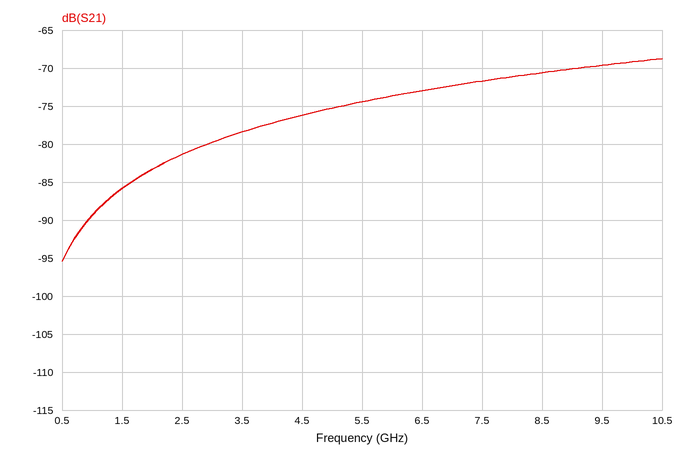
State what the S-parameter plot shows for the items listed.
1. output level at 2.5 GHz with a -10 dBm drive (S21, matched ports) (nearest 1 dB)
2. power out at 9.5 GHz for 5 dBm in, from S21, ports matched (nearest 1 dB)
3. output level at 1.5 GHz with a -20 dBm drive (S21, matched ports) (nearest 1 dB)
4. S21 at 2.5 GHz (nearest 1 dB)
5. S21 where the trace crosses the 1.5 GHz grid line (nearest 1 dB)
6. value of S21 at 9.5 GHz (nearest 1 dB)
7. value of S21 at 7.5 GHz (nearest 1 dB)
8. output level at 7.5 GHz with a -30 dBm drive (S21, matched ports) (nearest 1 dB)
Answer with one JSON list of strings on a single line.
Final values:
["-91 dBm", "-65 dBm", "-106 dBm", "-81 dB", "-86 dB", "-70 dB", "-72 dB", "-102 dBm"]
